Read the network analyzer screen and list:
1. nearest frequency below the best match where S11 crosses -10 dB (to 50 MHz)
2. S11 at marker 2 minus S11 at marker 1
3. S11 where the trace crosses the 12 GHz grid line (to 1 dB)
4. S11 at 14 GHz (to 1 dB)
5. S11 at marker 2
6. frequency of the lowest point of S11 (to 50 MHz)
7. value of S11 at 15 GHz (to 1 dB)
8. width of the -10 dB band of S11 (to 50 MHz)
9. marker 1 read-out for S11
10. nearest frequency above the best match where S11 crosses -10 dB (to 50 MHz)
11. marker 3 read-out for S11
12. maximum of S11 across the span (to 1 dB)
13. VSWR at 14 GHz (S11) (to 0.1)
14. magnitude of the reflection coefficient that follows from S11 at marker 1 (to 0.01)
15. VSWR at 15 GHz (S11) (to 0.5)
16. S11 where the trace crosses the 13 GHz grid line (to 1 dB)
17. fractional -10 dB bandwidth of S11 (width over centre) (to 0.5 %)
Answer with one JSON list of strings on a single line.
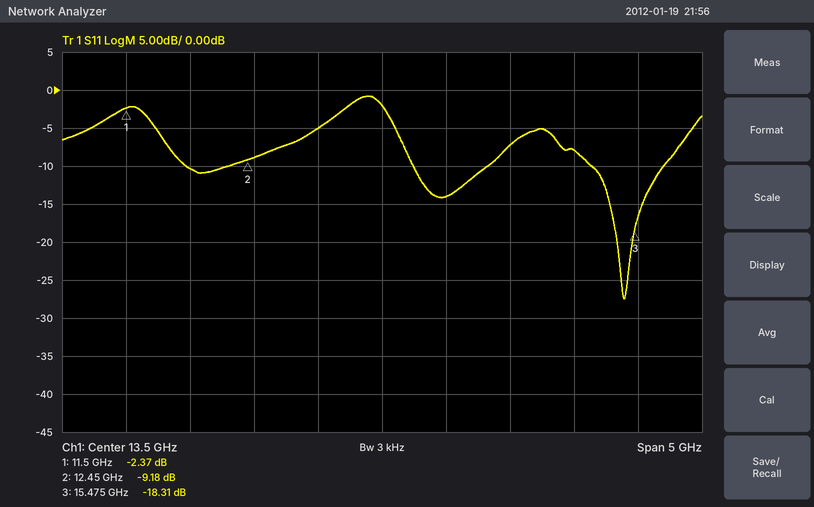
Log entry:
["15.15 GHz", "-6.81 dB", "-10 dB", "-14 dB", "-9.18 dB", "15.40 GHz", "-8 dB", "550 MHz", "-2.37 dB", "15.70 GHz", "-18.31 dB", "-1 dB", "1.5", "0.76", "2.5", "-5 dB", "3.5 %"]
